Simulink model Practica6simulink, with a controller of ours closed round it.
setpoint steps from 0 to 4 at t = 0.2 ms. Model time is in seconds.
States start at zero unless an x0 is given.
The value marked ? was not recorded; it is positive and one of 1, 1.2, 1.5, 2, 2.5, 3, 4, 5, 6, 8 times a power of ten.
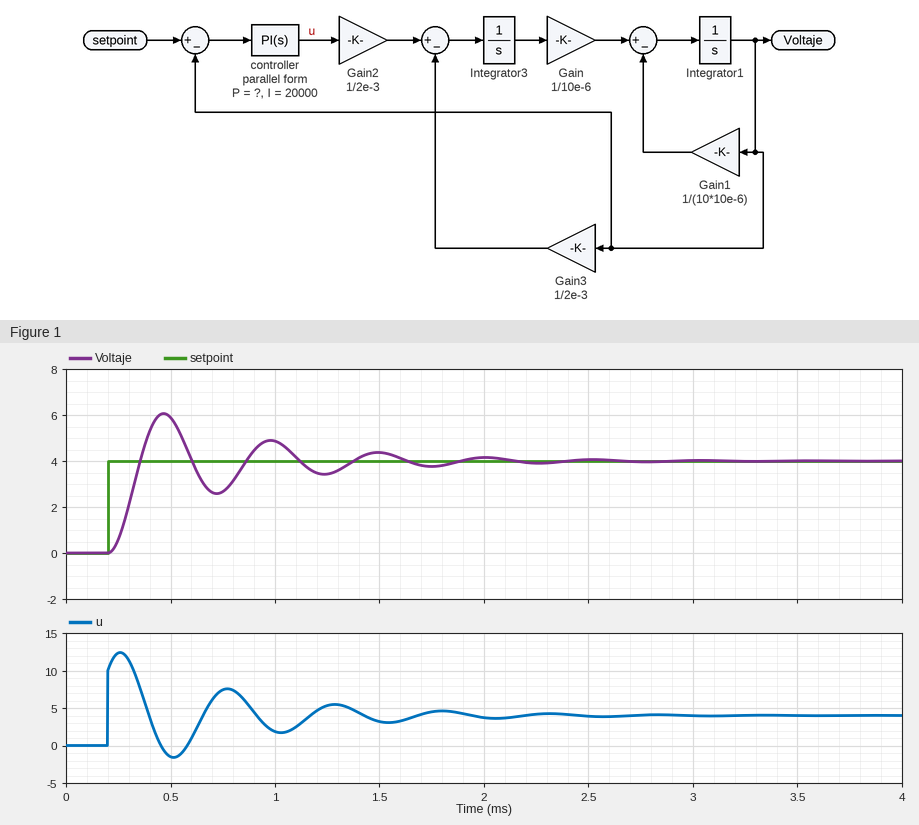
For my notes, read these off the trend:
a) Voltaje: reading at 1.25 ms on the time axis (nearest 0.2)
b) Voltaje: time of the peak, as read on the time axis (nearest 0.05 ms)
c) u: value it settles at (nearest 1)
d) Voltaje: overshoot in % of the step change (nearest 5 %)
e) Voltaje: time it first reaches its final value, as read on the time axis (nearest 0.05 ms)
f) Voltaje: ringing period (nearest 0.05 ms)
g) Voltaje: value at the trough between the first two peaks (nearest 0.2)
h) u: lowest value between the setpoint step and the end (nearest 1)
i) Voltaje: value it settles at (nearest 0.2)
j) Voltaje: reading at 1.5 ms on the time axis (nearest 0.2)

3.4
0.45 ms
4
50 %
0.35 ms
0.50 ms
2.6
-2
4.0
4.4
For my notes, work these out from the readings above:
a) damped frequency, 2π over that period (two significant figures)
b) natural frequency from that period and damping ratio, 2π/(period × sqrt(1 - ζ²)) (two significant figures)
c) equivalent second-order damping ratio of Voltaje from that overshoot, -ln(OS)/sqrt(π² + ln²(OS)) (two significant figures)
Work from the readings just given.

13 rad/ms
13 rad/ms
0.22
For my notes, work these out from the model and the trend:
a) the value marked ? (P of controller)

2.5
